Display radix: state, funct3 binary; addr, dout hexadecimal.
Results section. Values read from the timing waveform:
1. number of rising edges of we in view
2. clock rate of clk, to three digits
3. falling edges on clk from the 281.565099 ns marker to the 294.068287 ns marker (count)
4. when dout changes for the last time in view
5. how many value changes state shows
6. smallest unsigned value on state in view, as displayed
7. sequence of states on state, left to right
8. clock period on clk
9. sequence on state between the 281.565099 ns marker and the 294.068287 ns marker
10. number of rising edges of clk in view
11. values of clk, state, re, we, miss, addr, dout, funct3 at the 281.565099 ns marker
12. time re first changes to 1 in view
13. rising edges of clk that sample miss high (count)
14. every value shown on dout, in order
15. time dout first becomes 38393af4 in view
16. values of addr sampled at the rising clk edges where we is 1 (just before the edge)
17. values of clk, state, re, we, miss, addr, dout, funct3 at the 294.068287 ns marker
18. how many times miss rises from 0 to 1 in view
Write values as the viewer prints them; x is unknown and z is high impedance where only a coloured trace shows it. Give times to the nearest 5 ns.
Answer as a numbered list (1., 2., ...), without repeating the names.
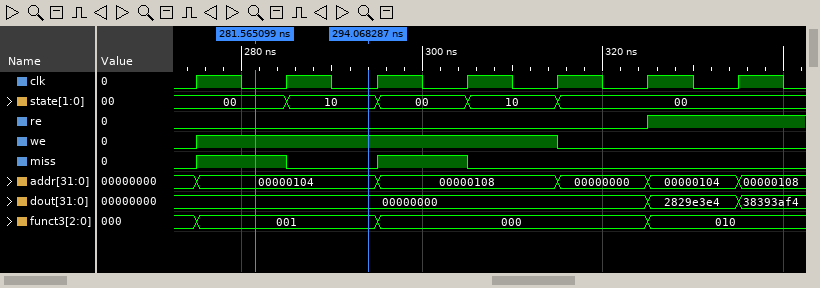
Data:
1. 1
2. 100 MHz
3. 1
4. 335 ns
5. 4
6. 00
7. 00, 10, 00, 10, 00
8. 10 ns
9. 00, 10
10. 7
11. clk=0, state=00, re=0, we=1, miss=1, addr=00000104, dout=00000000, funct3=001
12. 325 ns
13. 2
14. 00000000, 2829e3e4, 38393af4
15. 335 ns
16. 00000104, 00000104, 00000108, 00000108
17. clk=0, state=10, re=0, we=1, miss=0, addr=00000104, dout=00000000, funct3=001
18. 2
